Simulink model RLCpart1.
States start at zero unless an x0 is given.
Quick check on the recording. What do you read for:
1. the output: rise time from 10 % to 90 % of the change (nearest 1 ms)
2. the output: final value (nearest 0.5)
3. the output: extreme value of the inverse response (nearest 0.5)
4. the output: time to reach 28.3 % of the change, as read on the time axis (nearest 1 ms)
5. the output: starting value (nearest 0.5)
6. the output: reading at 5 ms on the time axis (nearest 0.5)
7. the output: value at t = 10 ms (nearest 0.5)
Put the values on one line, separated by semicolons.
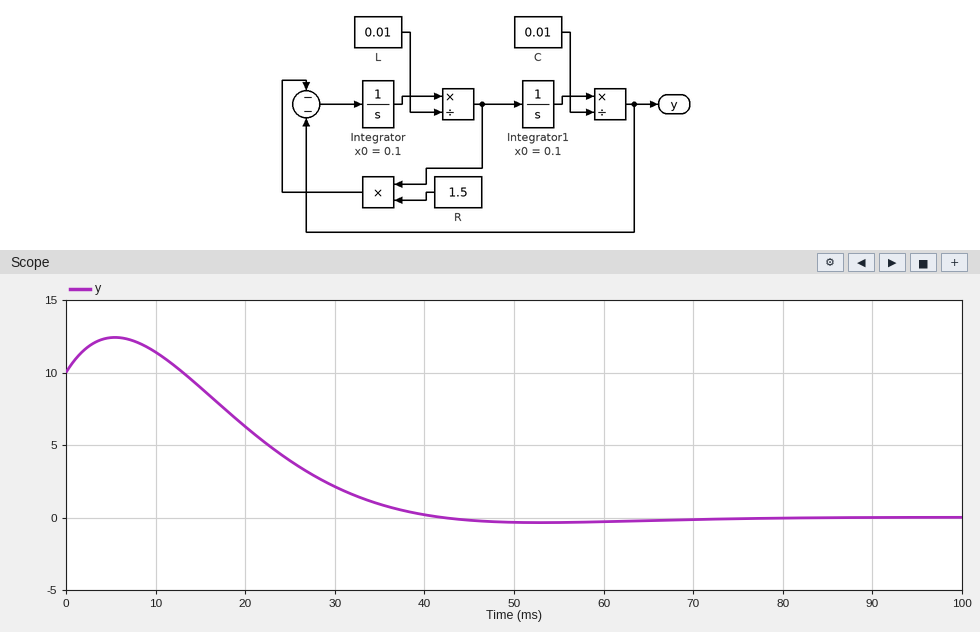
20 ms; 0.0; 12.5; 18 ms; 10.0; 12.5; 11.5
